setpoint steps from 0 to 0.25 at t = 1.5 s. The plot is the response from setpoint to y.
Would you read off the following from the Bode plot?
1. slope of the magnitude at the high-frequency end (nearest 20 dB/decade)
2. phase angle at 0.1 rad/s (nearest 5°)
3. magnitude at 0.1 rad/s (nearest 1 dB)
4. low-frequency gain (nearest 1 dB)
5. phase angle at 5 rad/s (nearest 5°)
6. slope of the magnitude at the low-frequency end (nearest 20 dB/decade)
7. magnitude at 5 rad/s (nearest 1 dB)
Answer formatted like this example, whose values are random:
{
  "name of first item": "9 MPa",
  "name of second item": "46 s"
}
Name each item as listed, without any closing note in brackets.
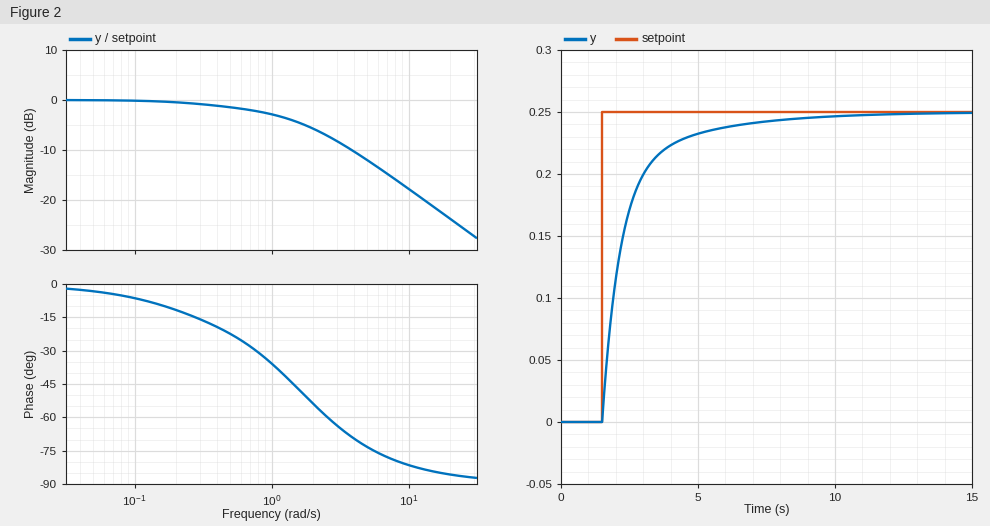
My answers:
{
  "slope of the magnitude at the high-frequency end": "-20 dB/decade",
  "phase angle at 0.1 rad/s": "-5°",
  "magnitude at 0.1 rad/s": "0 dB",
  "low-frequency gain": "0 dB",
  "phase angle at 5 rad/s": "-75°",
  "slope of the magnitude at the low-frequency end": "0 dB/decade",
  "magnitude at 5 rad/s": "-12 dB"
}
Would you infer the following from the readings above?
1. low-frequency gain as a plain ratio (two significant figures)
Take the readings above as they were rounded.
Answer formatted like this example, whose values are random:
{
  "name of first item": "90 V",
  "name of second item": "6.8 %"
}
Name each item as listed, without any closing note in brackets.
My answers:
{
  "low-frequency gain as a plain ratio": "1.0"
}
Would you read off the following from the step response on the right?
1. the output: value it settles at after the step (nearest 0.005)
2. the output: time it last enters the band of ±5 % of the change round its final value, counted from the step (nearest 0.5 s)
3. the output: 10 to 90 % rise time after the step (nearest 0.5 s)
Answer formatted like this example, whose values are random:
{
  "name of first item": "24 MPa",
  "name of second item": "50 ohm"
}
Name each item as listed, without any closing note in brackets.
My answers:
{
  "the output: value it settles at after the step": "0.250",
  "the output: time it last enters the band of ±5 % of the change round its final value, counted from the step": "4.5 s",
  "the output: 10 to 90 % rise time after the step": "2.5 s"
}
